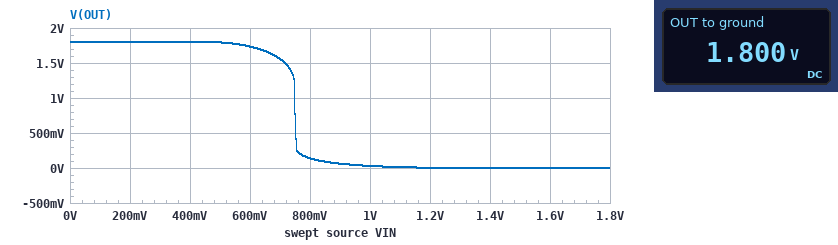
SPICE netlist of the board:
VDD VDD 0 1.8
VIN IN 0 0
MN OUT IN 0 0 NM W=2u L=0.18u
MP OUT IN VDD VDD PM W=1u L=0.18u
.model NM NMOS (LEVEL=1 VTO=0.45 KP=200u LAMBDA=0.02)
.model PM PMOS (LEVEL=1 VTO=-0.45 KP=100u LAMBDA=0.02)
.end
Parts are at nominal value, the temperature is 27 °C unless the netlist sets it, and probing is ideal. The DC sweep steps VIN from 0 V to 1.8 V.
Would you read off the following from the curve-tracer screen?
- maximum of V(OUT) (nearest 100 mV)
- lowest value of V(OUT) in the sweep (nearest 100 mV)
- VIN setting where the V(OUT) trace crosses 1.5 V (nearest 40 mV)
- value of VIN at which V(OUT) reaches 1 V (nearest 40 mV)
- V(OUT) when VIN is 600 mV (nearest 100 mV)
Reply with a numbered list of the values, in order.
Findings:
1. 1.8 V
2. 0 V
3. 720 mV
4. 760 mV
5. 1.7 V
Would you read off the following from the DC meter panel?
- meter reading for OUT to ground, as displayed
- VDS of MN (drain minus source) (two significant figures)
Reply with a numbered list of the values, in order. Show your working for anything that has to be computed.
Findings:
1. 1.800 V
2. 1.8 V = 1.8 V
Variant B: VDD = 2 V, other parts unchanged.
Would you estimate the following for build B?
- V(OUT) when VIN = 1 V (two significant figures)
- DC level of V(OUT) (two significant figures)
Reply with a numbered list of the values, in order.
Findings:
1. 77 mV
2. 2.0 V
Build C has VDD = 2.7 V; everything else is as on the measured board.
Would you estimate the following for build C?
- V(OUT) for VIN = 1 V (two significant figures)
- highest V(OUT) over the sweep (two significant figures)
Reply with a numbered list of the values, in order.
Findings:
1. 2.0 V
2. 2.7 V
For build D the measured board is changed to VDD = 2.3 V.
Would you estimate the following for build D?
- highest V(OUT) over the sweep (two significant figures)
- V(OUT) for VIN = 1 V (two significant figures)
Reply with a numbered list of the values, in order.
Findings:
1. 2.3 V
2. 210 mV
